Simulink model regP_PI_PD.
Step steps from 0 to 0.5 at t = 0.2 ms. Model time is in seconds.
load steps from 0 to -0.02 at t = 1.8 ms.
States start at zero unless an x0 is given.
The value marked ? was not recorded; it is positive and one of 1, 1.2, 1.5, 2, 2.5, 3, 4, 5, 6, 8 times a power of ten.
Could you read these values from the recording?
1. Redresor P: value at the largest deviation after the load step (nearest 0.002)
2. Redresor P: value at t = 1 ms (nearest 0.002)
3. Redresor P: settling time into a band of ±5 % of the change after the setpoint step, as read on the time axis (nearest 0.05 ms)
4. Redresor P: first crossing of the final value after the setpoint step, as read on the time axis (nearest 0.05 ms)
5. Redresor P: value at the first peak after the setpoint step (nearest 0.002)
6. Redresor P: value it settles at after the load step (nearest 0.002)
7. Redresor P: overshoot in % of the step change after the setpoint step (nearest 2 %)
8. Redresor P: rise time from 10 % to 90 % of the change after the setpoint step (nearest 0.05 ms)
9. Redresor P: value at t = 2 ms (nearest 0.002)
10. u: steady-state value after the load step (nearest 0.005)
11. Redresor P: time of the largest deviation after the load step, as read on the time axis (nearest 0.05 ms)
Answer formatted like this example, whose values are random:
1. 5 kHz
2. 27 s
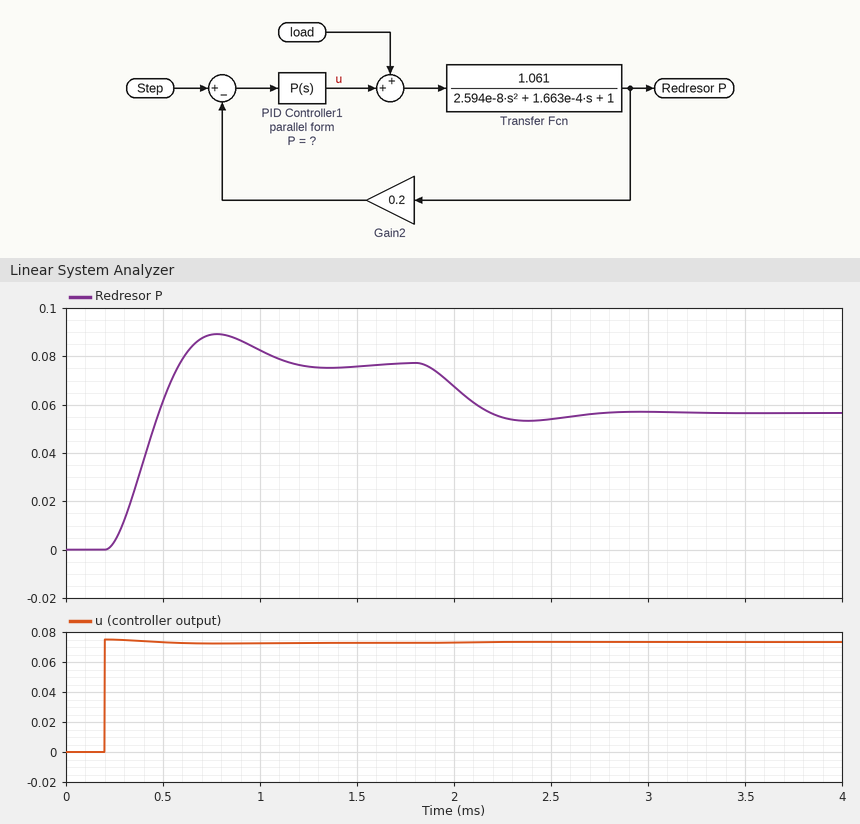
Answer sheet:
1. 0.054
2. 0.082
3. 1.05 ms
4. 0.60 ms
5. 0.090
6. 0.056
7. 16 %
8. 0.25 ms
9. 0.068
10. 0.075
11. 2.40 ms
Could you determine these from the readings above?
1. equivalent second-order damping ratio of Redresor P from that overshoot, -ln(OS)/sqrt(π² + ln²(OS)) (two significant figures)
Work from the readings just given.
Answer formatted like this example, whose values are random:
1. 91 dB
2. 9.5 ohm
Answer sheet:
1. 0.50
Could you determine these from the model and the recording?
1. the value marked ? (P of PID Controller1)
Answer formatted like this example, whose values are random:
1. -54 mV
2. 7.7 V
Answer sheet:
1. 0.15
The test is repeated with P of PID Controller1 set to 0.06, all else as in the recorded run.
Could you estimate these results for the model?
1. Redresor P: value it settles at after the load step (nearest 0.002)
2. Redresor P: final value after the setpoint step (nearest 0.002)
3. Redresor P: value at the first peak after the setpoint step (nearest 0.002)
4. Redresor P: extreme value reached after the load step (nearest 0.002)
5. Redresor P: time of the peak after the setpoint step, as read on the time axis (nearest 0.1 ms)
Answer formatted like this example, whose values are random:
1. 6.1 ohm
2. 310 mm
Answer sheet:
1. 0.010
2. 0.032
3. 0.036
4. 0.008
5. 0.8 ms
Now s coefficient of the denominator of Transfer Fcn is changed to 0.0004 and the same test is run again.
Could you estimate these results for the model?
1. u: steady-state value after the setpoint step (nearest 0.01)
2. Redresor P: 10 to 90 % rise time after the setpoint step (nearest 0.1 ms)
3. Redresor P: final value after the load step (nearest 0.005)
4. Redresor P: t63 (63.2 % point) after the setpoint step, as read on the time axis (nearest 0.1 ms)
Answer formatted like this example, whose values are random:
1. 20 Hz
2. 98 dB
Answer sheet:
1. 0.07
2. 0.7 ms
3. 0.055
4. 0.6 ms
